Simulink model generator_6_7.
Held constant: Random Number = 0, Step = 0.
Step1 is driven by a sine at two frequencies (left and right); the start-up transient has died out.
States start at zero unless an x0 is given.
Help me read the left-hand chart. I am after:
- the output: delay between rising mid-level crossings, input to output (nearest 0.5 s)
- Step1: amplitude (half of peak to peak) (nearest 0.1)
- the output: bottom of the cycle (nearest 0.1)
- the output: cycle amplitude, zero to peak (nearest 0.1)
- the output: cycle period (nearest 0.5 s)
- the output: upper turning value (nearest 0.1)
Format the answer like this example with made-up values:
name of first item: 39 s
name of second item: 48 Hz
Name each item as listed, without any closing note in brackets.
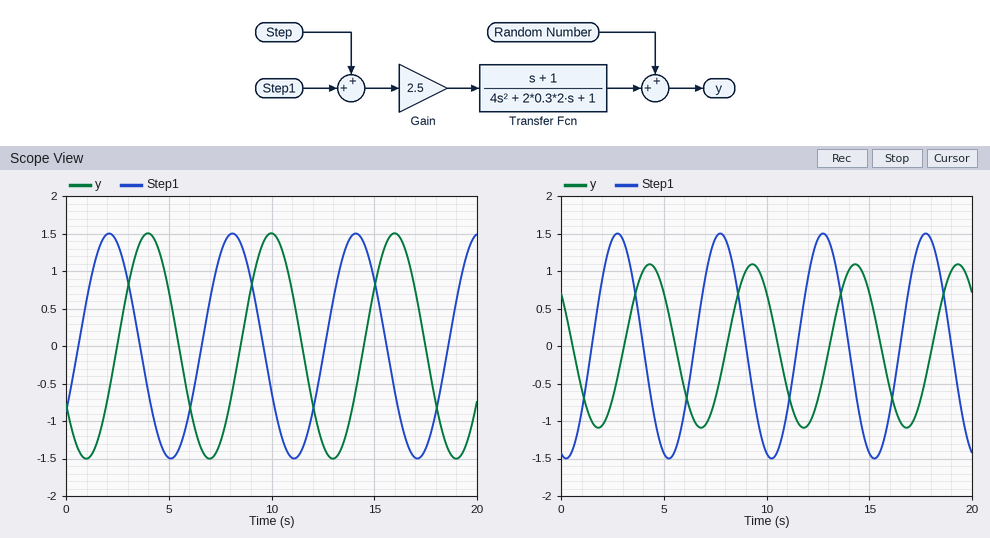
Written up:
the output: delay between rising mid-level crossings, input to output: 2.0 s
Step1: amplitude (half of peak to peak): 1.5
the output: bottom of the cycle: -1.5
the output: cycle amplitude, zero to peak: 1.5
the output: cycle period: 6.0 s
the output: upper turning value: 1.5
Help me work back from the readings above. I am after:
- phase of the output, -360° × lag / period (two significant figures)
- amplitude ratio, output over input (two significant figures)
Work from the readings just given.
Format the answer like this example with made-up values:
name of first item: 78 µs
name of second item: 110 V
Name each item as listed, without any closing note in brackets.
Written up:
phase of the output, -360° × lag / period: -120°
amplitude ratio, output over input: 1.0
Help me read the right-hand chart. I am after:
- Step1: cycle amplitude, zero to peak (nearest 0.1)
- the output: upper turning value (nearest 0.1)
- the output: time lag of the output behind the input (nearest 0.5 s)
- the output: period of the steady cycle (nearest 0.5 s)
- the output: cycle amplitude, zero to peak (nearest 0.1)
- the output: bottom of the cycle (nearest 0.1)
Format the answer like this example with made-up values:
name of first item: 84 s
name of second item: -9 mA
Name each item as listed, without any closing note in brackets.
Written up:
Step1: cycle amplitude, zero to peak: 1.5
the output: upper turning value: 1.1
the output: time lag of the output behind the input: 1.5 s
the output: period of the steady cycle: 5.0 s
the output: cycle amplitude, zero to peak: 1.1
the output: bottom of the cycle: -1.1
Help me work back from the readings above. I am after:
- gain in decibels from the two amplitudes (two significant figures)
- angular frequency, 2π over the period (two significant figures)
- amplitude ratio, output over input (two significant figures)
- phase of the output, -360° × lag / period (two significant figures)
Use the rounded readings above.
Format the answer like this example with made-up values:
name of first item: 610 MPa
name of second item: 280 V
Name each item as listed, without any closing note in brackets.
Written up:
gain in decibels from the two amplitudes: -2.7 dB
angular frequency, 2π over the period: 1.3 rad/s
amplitude ratio, output over input: 0.73
phase of the output, -360° × lag / period: -110°
